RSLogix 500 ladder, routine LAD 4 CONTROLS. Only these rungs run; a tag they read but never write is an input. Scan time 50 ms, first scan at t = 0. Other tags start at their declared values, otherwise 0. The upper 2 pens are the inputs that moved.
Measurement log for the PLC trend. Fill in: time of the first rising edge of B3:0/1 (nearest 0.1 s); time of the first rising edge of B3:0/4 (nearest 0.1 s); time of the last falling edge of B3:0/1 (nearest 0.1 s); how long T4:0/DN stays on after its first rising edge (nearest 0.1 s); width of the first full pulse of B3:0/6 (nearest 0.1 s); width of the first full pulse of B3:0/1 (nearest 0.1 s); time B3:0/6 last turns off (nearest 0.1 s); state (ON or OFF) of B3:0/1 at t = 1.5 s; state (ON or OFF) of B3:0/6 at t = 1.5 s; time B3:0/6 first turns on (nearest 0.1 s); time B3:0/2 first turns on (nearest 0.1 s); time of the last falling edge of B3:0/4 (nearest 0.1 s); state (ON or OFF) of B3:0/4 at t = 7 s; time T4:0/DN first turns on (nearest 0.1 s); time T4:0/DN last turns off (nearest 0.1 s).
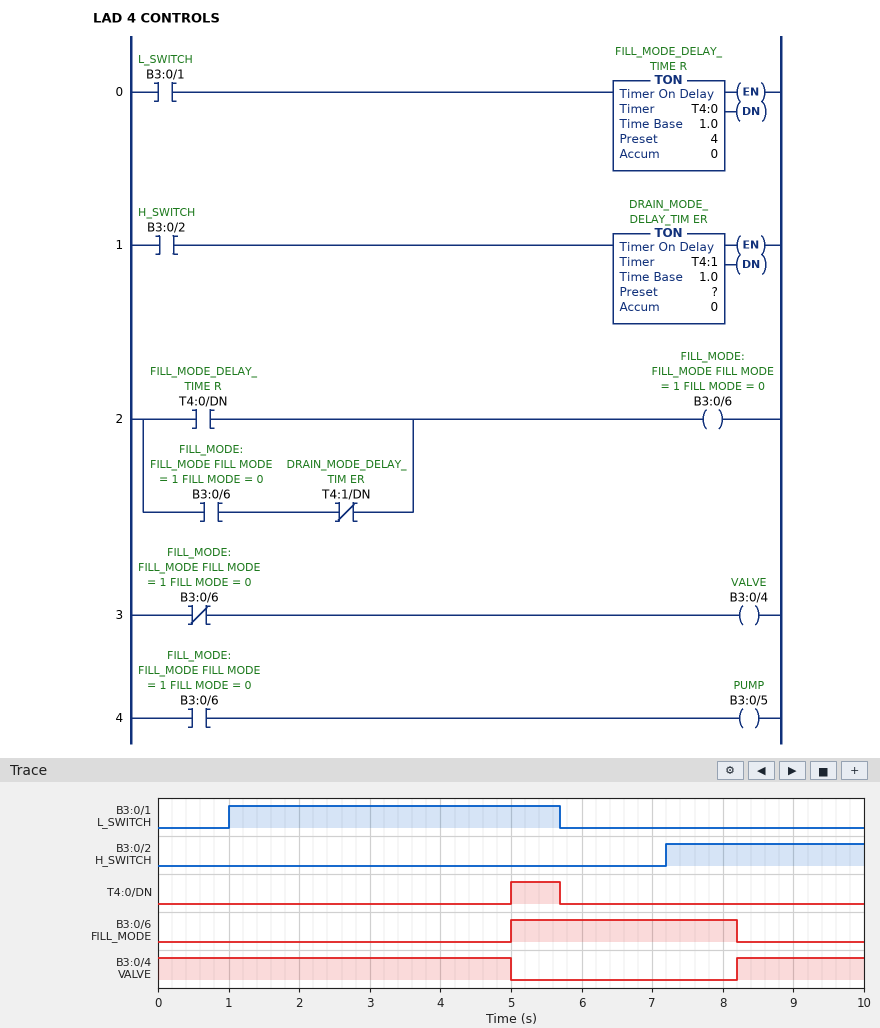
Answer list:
1.0 s
8.2 s
5.7 s
0.7 s
3.2 s
4.7 s
8.2 s
ON
OFF
5.0 s
7.2 s
5.0 s
OFF
5.0 s
5.7 s
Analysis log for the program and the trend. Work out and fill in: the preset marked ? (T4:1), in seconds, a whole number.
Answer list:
1 s
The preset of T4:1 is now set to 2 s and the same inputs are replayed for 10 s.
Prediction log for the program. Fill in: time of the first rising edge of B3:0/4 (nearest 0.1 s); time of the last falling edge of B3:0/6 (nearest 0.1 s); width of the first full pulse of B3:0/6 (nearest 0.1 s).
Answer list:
9.2 s
9.2 s
4.2 s
